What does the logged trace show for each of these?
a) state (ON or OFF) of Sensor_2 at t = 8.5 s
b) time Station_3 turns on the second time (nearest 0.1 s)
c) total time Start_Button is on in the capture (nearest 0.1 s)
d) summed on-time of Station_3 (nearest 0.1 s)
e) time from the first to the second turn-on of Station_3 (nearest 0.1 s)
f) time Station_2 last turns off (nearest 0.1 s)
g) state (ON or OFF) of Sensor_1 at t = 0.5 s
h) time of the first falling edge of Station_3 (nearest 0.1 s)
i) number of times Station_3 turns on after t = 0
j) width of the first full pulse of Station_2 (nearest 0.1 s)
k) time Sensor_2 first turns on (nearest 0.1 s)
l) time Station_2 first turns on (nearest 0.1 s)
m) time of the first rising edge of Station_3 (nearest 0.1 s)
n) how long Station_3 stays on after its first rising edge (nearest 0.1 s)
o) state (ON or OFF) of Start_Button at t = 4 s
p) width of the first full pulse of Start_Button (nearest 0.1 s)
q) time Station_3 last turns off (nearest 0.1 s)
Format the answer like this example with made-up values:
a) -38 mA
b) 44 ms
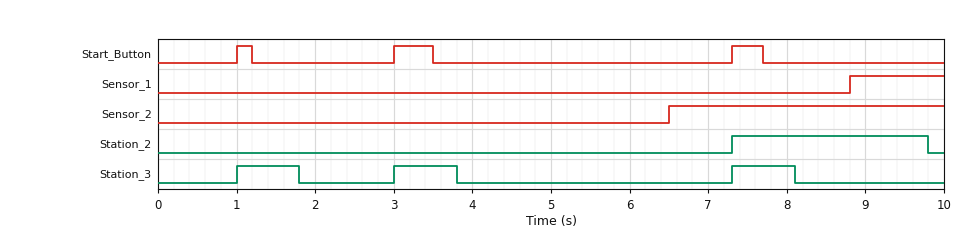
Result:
a) ON
b) 3.0 s
c) 1.1 s
d) 2.4 s
e) 2.0 s
f) 9.8 s
g) OFF
h) 1.8 s
i) 3
j) 2.5 s
k) 6.5 s
l) 7.3 s
m) 1.0 s
n) 0.8 s
o) OFF
p) 0.2 s
q) 8.1 s
